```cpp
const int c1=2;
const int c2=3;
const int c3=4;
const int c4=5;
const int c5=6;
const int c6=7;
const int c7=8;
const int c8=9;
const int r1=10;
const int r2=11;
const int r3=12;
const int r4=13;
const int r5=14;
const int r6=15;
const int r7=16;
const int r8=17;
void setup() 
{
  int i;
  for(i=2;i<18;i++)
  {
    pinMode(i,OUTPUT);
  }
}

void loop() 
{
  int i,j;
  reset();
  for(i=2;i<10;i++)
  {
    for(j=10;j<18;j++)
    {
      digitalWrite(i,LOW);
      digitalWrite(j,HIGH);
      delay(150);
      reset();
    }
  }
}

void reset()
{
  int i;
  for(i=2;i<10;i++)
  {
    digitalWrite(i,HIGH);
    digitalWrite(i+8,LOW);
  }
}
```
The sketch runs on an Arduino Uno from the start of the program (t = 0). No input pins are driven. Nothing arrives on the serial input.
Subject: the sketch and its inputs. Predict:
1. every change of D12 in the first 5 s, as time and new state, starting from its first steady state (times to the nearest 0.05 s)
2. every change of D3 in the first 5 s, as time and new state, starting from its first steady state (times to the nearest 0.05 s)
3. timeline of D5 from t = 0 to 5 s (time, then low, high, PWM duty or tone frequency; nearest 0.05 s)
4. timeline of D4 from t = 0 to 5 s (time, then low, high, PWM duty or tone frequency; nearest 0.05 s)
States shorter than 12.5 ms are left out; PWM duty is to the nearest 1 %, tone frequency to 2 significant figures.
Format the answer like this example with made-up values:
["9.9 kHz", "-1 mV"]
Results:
["0 s low; 0.3 s high; 0.45 s low; 1.5 s high; 1.65 s low; 2.7 s high; 2.85 s low; 3.9 s high; 4.05 s low", "0 s high; 1.2 s low; 2.4 s high", "0 s high; 3.6 s low; 4.8 s high", "0 s high; 2.4 s low; 3.6 s high"]
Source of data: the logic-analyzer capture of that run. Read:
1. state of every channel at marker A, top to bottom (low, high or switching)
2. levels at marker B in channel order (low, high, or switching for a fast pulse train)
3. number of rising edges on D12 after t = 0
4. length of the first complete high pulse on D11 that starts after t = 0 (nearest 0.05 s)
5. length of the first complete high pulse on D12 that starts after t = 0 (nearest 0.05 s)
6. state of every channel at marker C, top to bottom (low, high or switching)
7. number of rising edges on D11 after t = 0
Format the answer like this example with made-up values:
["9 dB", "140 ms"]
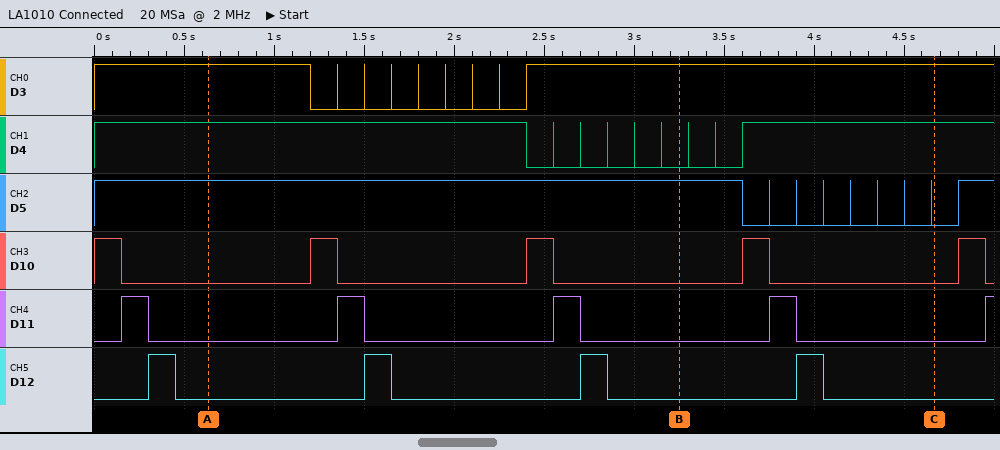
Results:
["D3 high, D4 high, D5 high, D10 low, D11 low, D12 low", "D3 high, D4 low, D5 high, D10 low, D11 low, D12 low", "4", "0.15 s", "0.15 s", "D3 high, D4 high, D5 low, D10 low, D11 low, D12 low", "5"]
